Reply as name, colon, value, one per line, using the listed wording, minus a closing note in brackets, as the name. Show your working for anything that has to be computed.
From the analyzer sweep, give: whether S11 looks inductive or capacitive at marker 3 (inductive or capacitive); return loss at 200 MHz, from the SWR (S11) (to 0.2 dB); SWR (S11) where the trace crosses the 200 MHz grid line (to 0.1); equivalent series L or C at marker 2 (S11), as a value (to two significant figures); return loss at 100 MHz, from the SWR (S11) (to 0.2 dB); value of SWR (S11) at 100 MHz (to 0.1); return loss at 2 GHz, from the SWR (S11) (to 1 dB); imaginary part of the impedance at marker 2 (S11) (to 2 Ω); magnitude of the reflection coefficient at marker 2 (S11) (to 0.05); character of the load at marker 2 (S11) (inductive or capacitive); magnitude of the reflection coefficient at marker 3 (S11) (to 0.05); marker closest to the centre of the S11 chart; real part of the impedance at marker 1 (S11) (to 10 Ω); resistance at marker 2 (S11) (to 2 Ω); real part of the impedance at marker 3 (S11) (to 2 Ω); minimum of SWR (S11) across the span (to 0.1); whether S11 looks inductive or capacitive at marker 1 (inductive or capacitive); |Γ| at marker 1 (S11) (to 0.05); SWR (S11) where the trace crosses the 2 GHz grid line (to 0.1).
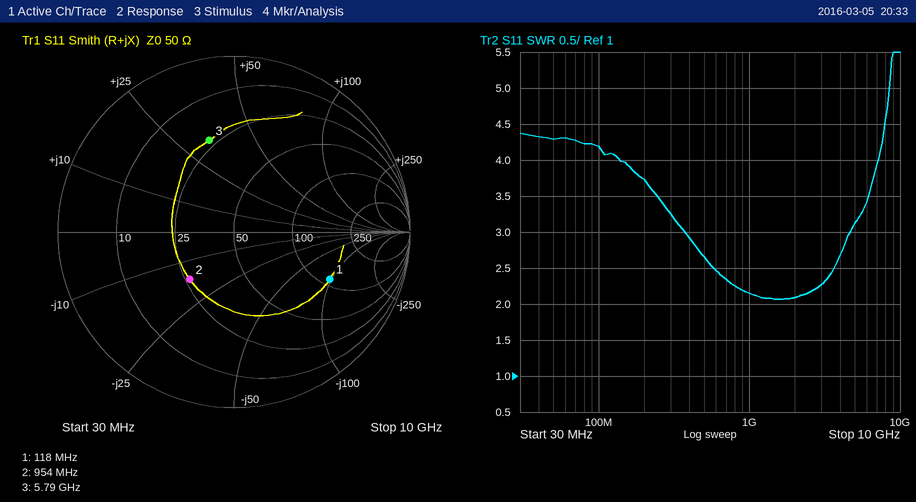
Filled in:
whether S11 looks inductive or capacitive at marker 3: inductive
return loss at 200 MHz, from the SWR (S11): −20 log10((3.7 − 1)/(3.7 + 1)) ≈ 4.8 dB
SWR (S11) where the trace crosses the 200 MHz grid line: 3.7
equivalent series L or C at marker 2 (S11), as a value: C = 1/(2π × 954 MHz × 16 Ω) ≈ 10 pF
return loss at 100 MHz, from the SWR (S11): −20 log10((4.2 − 1)/(4.2 + 1)) ≈ 4.2 dB
value of SWR (S11) at 100 MHz: 4.2
return loss at 2 GHz, from the SWR (S11): −20 log10((2.1 − 1)/(2.1 + 1)) ≈ 9 dB
imaginary part of the impedance at marker 2 (S11): -16 Ω
magnitude of the reflection coefficient at marker 2 (S11): 0.35
character of the load at marker 2 (S11): capacitive
magnitude of the reflection coefficient at marker 3 (S11): 0.55
marker closest to the centre of the S11 chart: marker 2
real part of the impedance at marker 1 (S11): 110 Ω
resistance at marker 2 (S11): 26 Ω
real part of the impedance at marker 3 (S11): 22 Ω
minimum of SWR (S11) across the span: 2.1
whether S11 looks inductive or capacitive at marker 1: capacitive
|Γ| at marker 1 (S11): 0.60
SWR (S11) where the trace crosses the 2 GHz grid line: 2.1
